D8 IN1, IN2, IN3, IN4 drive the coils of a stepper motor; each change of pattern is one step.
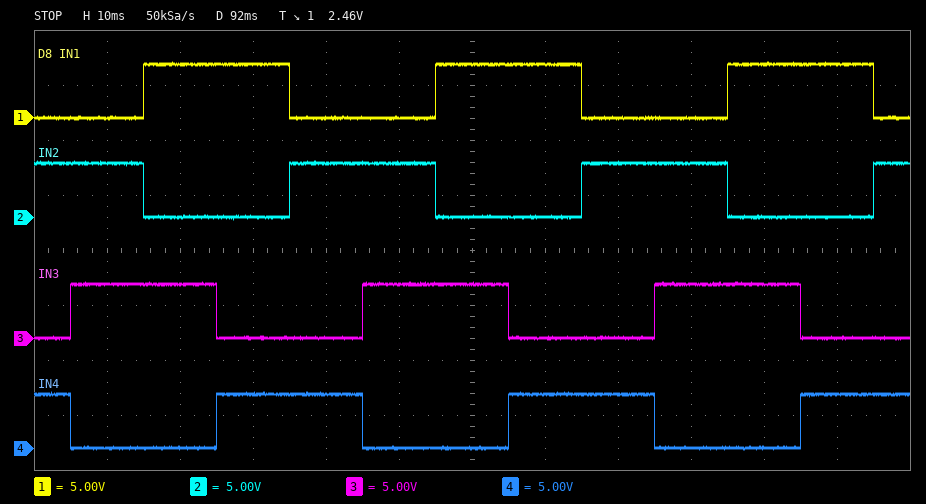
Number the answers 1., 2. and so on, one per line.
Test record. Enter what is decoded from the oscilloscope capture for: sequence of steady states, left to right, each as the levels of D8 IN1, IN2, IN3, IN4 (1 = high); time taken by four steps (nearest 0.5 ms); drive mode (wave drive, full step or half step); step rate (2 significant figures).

1. 0101 0110 1010 1001 0101 0110 1010 1001 0101 0110 1010 1001 0101
2. 40.0 ms
3. full step
4. 100 steps/s
